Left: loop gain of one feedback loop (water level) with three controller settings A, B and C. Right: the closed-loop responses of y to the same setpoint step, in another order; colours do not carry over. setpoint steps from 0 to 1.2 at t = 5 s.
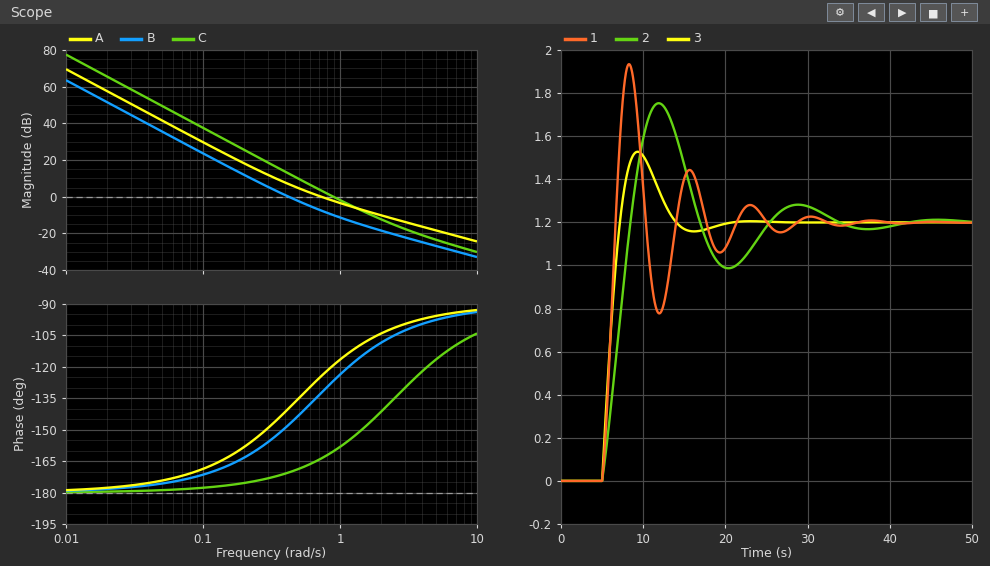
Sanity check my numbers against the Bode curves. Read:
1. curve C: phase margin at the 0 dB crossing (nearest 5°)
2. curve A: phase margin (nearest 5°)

20°
55°
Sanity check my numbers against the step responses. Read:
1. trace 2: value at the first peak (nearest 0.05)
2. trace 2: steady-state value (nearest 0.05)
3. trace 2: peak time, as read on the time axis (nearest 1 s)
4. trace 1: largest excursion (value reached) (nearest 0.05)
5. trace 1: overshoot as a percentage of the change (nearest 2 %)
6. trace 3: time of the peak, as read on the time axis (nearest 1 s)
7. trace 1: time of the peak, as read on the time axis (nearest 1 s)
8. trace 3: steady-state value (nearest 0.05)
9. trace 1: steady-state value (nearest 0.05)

1.75
1.20
12 s
1.95
62 %
9 s
8 s
1.20
1.20
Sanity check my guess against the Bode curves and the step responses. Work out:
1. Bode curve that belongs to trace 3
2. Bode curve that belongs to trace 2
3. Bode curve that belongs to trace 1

A
B
C
